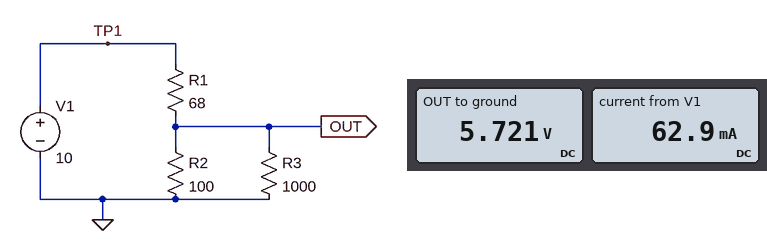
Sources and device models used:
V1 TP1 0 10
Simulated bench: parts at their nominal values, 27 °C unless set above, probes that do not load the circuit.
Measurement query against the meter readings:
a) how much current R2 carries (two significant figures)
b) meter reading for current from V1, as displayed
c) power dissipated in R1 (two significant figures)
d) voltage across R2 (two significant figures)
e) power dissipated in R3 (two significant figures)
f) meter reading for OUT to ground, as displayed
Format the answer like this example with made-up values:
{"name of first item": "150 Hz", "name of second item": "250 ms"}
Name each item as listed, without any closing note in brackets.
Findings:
{"how much current R2 carries": "57 mA", "meter reading for current from V1, as displayed": "62.9 mA", "power dissipated in R1": "270 mW", "voltage across R2": "5.7 V", "power dissipated in R3": "33 mW", "meter reading for OUT to ground, as displayed": "5.721 V"}
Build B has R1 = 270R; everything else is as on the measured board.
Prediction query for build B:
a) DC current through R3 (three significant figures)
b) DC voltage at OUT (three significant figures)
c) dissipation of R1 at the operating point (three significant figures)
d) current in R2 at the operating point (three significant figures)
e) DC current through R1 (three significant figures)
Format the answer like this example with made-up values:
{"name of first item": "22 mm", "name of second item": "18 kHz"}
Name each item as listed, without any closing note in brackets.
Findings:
{"DC current through R3": "2.52 mA", "DC voltage at OUT": "2.52 V", "dissipation of R1 at the operating point": "207 mW", "current in R2 at the operating point": "25.2 mA", "DC current through R1": "27.7 mA"}
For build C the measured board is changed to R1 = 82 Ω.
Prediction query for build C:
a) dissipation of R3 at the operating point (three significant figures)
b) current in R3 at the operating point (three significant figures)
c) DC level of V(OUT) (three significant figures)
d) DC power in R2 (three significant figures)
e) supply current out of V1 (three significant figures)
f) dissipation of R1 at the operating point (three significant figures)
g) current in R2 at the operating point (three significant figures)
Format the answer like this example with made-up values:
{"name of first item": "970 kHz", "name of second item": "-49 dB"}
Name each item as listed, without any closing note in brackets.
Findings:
{"dissipation of R3 at the operating point": "27.6 mW", "current in R3 at the operating point": "5.26 mA", "DC level of V(OUT)": "5.26 V", "DC power in R2": "276 mW", "supply current out of V1": "57.8 mA", "dissipation of R1 at the operating point": "274 mW", "current in R2 at the operating point": "52.6 mA"}
